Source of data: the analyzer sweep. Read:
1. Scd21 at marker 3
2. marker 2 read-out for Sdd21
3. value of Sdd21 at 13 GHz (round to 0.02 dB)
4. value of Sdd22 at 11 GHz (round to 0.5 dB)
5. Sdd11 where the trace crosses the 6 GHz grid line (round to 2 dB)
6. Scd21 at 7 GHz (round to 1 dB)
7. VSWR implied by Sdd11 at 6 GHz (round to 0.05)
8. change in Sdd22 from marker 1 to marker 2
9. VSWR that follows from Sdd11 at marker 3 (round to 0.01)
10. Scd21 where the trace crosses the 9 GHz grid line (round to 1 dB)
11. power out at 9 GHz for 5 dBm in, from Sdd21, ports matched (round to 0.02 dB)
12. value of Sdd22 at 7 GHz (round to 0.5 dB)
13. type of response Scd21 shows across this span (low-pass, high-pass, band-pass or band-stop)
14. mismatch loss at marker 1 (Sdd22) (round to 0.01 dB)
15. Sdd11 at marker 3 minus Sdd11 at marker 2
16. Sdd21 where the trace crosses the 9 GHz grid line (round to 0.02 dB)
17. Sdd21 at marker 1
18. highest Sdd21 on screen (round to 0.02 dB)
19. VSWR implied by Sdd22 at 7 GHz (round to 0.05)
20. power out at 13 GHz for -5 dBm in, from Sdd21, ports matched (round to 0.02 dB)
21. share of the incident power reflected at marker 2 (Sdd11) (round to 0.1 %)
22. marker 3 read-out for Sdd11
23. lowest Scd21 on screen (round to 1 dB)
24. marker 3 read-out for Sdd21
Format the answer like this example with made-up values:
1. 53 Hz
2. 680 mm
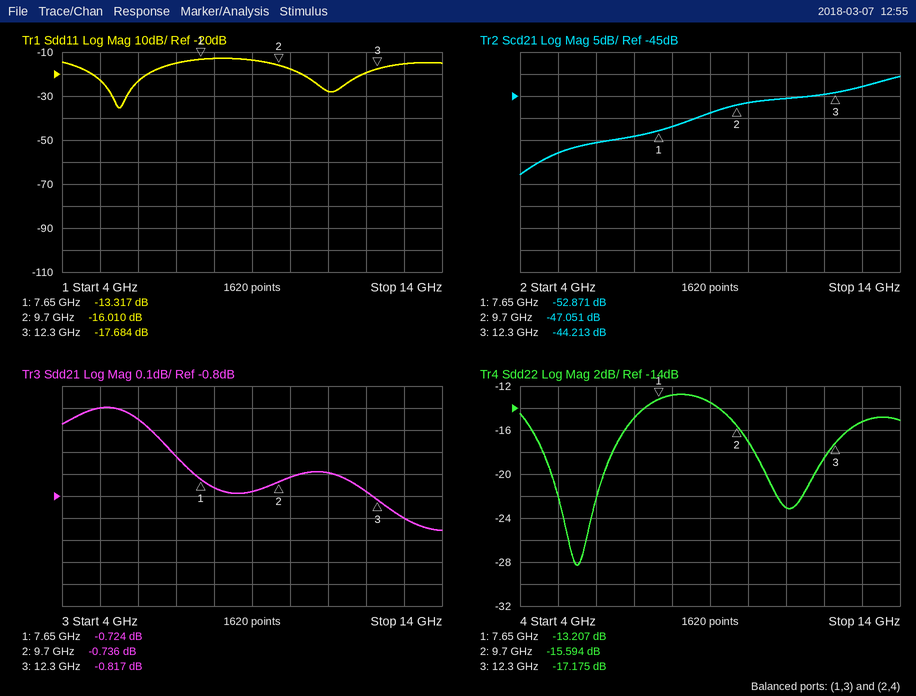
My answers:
1. -44.213 dB
2. -0.736 dB
3. -0.90 dB
4. -23.0 dB
5. -24 dB
6. -54 dB
7. 1.15
8. -2.387 dB
9. 1.30
10. -49 dB
11. 4.22 dBm
12. -15.0 dB
13. high-pass
14. 0.21 dB
15. -1.674 dB
16. -0.78 dB
17. -0.724 dB
18. -0.40 dB
19. 1.45
20. -5.90 dBm
21. 2.5 %
22. -17.684 dB
23. -63 dB
24. -0.817 dB
